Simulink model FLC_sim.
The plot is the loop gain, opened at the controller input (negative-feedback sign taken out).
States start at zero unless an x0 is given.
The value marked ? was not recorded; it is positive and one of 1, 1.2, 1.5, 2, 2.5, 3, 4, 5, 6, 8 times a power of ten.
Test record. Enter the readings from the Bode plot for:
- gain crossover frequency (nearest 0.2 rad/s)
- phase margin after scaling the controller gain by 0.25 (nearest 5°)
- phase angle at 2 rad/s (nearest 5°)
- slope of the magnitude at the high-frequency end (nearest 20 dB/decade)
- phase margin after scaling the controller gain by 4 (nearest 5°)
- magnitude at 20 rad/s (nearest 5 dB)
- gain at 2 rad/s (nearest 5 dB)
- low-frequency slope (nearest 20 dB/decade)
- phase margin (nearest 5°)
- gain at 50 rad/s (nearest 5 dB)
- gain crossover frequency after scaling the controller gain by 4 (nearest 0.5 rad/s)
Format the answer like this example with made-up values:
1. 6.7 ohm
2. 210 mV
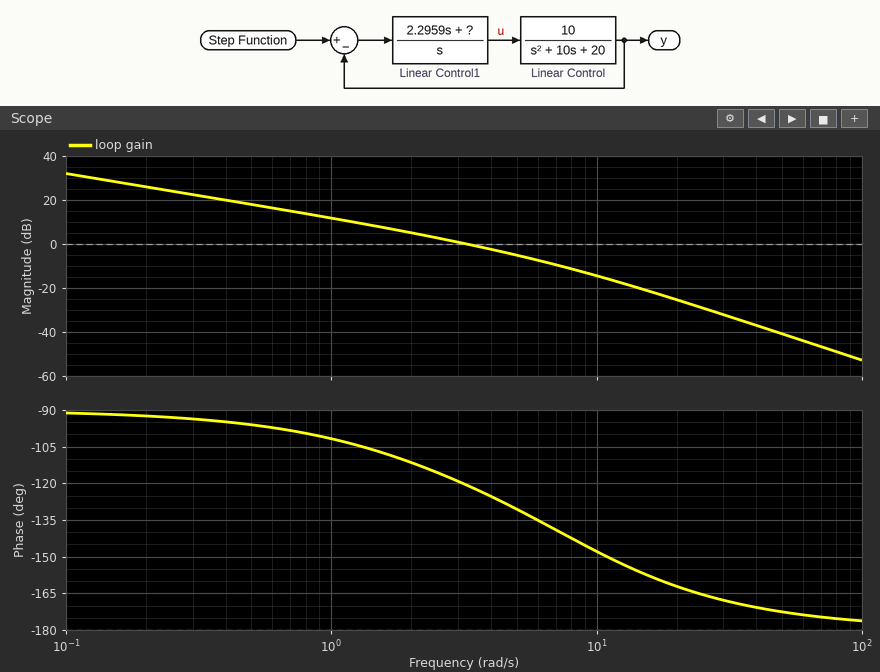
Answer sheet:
1. 3.2 rad/s
2. 80°
3. -110°
4. -40 dB/decade
5. 35°
6. -25 dB
7. 5 dB
8. -20 dB/decade
9. 60°
10. -40 dB
11. 8.5 rad/s
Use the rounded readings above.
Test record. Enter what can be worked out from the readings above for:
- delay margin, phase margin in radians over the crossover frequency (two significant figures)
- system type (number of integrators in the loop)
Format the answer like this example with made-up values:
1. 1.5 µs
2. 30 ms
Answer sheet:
1. 0.33 s
2. 1
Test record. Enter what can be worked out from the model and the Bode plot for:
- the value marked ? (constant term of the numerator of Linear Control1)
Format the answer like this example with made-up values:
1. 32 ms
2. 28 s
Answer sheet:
1. 8
